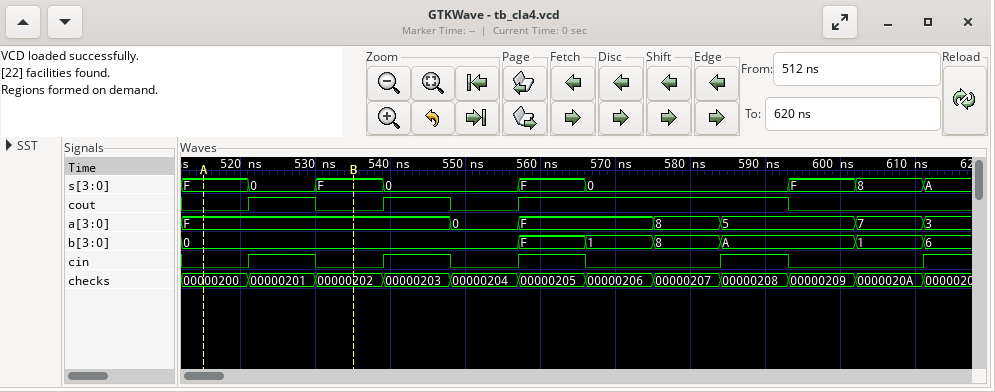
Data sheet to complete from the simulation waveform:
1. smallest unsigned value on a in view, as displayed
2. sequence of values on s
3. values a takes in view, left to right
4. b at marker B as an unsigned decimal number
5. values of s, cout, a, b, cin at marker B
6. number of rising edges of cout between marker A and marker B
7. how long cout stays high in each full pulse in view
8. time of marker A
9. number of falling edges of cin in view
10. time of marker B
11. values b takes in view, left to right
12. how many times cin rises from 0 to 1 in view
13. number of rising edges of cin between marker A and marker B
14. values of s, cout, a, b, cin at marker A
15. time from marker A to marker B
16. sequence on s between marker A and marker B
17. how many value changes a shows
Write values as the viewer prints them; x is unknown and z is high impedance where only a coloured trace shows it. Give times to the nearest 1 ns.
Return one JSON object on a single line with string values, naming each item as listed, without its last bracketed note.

{"smallest unsigned value on a in view, as displayed": "0", "sequence of values on s": "F, 0, F, 0, F, 0, F, 8, A", "values a takes in view, left to right": "F, 0, F, 8, 5, 7, 3", "b at marker B as an unsigned decimal number": "0", "values of s, cout, a, b, cin at marker B": "s=F, cout=0, a=F, b=0, cin=0", "number of rising edges of cout between marker A and marker B": "1", "how long cout stays high in each full pulse in view": "9 ns, 9 ns, 36 ns", "time of marker A": "515 ns", "number of falling edges of cin in view": "4", "time of marker B": "535 ns", "values b takes in view, left to right": "0, F, 1, 8, A, 1, 6", "how many times cin rises from 0 to 1 in view": "5", "number of rising edges of cin between marker A and marker B": "1", "values of s, cout, a, b, cin at marker A": "s=F, cout=0, a=F, b=0, cin=0", "time from marker A to marker B": "20 ns", "sequence on s between marker A and marker B": "F, 0, F", "how many value changes a shows": "6"}
